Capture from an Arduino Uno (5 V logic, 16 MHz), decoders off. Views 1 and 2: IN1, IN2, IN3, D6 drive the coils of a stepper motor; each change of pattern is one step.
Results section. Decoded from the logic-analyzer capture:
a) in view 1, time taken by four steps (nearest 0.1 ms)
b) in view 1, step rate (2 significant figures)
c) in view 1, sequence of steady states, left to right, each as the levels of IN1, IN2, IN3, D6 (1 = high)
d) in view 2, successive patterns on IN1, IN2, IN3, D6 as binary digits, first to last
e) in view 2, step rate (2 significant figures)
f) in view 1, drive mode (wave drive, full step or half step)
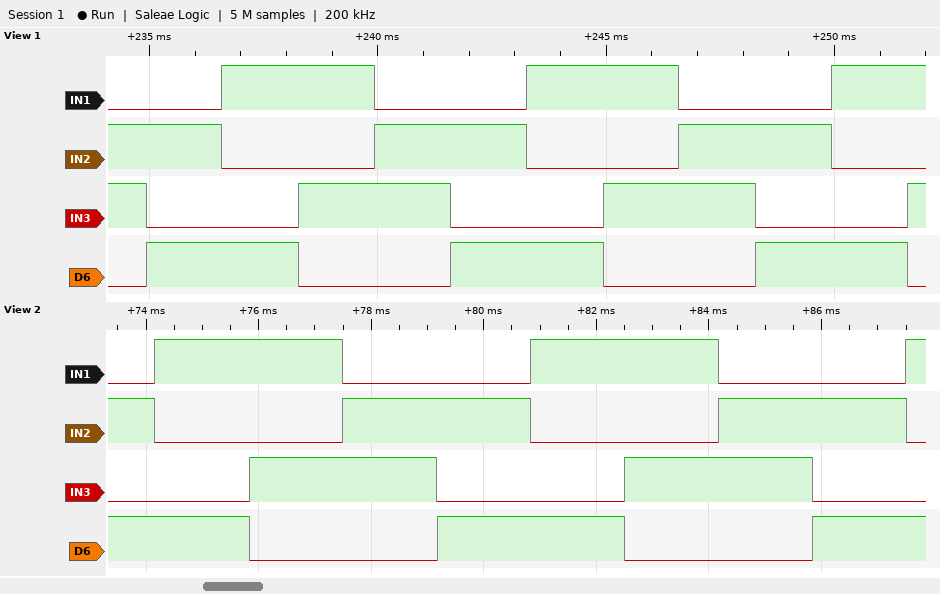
6.7 ms
600 steps/s
0110 0101 1001 1010 0110 0101 1001 1010 0110 0101 1001 1010
0101 1001 1010 0110 0101 1001 1010 0110 0101 1001
600 steps/s
full step
